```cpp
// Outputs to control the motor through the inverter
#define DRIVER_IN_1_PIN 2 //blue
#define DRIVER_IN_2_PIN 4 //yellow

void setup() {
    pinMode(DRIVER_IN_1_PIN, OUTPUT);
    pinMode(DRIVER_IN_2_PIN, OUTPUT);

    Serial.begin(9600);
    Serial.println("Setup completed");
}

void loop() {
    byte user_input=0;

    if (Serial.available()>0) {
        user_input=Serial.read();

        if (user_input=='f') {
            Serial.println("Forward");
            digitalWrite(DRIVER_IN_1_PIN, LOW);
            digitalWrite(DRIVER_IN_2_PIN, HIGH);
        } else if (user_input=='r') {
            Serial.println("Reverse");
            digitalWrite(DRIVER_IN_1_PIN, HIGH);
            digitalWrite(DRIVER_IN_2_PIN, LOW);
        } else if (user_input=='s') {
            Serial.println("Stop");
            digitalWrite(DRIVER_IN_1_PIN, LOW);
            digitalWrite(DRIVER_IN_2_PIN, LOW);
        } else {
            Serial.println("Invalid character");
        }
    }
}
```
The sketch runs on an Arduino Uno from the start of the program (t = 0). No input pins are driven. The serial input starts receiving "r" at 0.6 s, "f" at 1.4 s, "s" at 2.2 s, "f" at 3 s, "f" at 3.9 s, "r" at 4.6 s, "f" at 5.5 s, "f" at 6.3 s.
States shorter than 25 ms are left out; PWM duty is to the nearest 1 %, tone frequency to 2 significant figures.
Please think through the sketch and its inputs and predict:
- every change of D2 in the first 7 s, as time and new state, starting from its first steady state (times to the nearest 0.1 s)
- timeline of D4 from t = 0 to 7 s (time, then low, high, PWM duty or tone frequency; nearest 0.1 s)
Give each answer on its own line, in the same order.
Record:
0 s low; 0.6 s high; 1.4 s low; 4.6 s high; 5.5 s low
0 s low; 1.4 s high; 2.2 s low; 3 s high; 4.6 s low; 5.5 s high
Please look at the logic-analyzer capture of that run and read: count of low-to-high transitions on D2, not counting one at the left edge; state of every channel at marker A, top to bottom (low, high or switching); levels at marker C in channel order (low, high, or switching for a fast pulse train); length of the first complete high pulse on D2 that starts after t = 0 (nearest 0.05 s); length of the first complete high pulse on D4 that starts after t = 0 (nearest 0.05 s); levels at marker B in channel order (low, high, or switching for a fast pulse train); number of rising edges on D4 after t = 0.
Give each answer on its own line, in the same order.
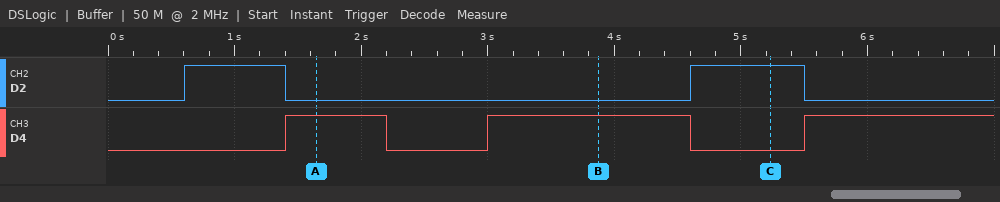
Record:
2
D2 low, D4 high
D2 high, D4 low
0.80 s
0.80 s
D2 low, D4 high
3
